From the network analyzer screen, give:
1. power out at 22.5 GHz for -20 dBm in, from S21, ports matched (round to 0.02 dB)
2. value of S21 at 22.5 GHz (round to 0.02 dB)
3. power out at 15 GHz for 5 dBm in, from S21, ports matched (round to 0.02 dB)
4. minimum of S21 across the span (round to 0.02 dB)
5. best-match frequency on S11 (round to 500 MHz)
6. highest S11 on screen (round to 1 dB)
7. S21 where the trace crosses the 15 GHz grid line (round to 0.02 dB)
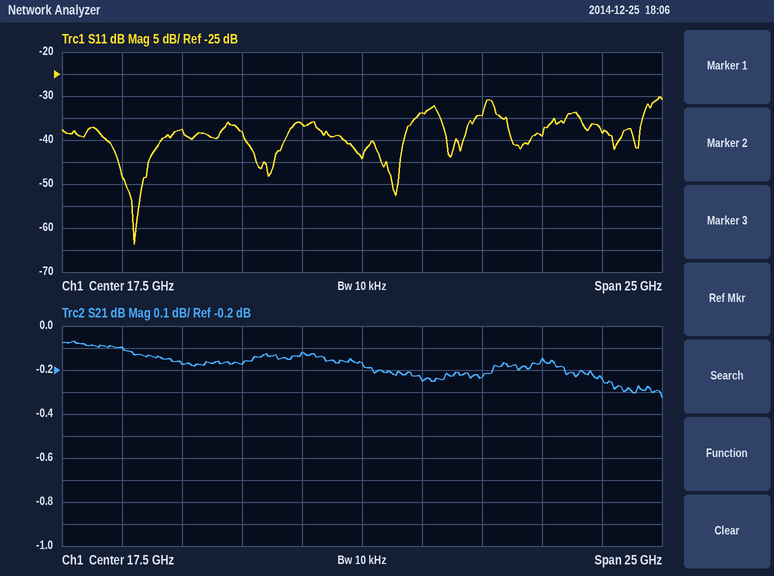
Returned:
-20.24 dBm
-0.24 dB
4.88 dBm
-0.32 dB
8.0 GHz
-30 dB
-0.12 dB
